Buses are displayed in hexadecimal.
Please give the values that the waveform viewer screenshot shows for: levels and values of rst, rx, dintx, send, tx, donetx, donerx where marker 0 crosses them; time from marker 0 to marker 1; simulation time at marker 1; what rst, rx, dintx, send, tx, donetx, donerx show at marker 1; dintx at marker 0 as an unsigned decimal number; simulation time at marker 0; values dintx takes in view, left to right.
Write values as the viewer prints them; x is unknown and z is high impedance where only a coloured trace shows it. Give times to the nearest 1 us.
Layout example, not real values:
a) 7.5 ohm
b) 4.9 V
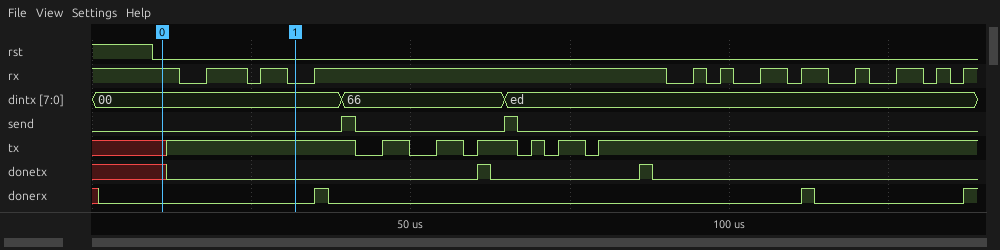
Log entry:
a) rst=0, rx=1, dintx=00, send=0, tx=x, donetx=x, donerx=0
b) 21 us
c) 32 us
d) rst=0, rx=0, dintx=00, send=0, tx=1, donetx=0, donerx=0
e) 0
f) 11 us
g) 00, 66, ed
